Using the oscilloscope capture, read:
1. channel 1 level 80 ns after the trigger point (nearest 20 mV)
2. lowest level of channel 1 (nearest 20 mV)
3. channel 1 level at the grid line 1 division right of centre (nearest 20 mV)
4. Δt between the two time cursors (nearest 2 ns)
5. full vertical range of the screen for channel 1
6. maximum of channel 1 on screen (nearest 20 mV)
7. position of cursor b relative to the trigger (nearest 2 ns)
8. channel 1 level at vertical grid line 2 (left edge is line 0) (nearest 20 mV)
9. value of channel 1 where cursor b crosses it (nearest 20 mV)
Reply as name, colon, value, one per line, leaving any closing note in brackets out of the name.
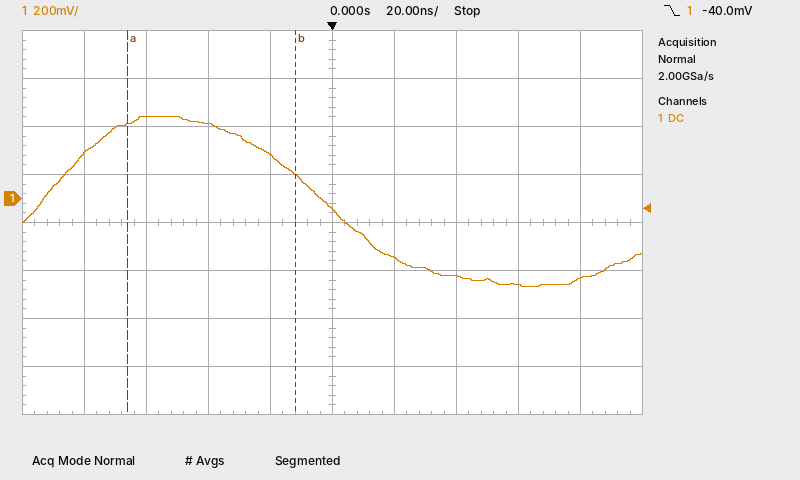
channel 1 level 80 ns after the trigger point: -340 mV
lowest level of channel 1: -360 mV
channel 1 level at the grid line 1 division right of centre: -240 mV
Δt between the two time cursors: 54 ns
full vertical range of the screen for channel 1: 1.6 V
maximum of channel 1 on screen: 340 mV
position of cursor b relative to the trigger: -12 ns
channel 1 level at vertical grid line 2 (left edge is line 0): 340 mV
value of channel 1 where cursor b crosses it: 100 mV
